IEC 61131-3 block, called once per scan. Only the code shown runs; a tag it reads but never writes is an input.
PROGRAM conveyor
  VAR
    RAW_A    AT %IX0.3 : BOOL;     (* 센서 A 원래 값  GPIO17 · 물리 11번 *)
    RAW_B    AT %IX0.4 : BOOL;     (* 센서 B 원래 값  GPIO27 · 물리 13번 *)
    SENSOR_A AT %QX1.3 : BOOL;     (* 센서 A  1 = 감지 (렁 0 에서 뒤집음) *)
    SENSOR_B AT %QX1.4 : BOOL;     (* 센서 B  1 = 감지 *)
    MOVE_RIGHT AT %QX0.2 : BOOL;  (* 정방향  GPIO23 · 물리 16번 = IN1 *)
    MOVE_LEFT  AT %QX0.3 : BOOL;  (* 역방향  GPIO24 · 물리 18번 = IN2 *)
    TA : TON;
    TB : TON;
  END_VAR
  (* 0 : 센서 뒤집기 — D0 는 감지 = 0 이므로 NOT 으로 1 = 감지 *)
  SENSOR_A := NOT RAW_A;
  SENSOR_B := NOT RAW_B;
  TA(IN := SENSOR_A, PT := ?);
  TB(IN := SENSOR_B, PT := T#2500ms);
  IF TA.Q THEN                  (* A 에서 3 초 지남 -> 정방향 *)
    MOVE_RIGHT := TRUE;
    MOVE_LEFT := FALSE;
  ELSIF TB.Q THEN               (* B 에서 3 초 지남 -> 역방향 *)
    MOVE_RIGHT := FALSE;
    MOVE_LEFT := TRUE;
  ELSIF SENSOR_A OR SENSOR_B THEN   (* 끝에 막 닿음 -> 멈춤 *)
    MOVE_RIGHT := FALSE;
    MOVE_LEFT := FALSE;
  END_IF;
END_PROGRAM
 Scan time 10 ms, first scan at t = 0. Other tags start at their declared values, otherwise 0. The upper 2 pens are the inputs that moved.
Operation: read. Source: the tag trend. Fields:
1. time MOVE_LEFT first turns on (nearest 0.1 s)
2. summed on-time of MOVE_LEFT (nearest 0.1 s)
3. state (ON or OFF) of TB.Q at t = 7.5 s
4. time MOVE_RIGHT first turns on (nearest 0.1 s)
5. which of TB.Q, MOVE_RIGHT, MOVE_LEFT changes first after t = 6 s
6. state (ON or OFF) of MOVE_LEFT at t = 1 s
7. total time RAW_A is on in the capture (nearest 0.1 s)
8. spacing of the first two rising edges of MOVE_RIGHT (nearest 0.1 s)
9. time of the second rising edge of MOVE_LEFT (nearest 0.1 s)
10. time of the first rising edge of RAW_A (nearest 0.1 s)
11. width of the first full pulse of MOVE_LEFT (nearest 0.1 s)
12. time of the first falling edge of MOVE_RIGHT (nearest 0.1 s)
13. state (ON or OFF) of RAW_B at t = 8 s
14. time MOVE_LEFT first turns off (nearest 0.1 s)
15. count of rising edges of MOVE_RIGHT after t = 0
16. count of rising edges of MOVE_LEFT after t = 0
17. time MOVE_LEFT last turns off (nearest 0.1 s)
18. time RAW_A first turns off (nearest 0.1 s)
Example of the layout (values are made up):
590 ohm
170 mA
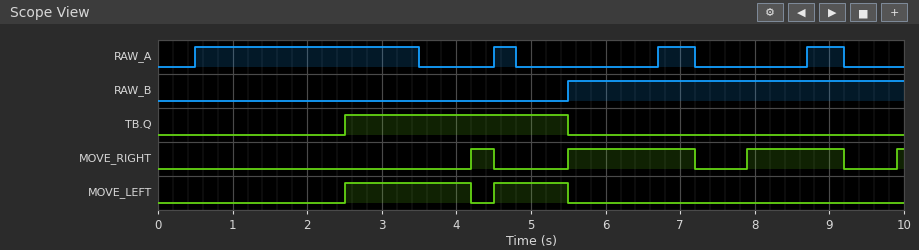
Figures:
2.5 s
2.7 s
OFF
4.2 s
MOVE_RIGHT
OFF
4.3 s
1.3 s
4.5 s
0.5 s
1.7 s
4.5 s
ON
4.2 s
4
2
5.5 s
3.5 s
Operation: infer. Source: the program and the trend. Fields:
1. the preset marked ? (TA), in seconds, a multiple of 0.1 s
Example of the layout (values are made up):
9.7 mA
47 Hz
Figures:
0.7 s
